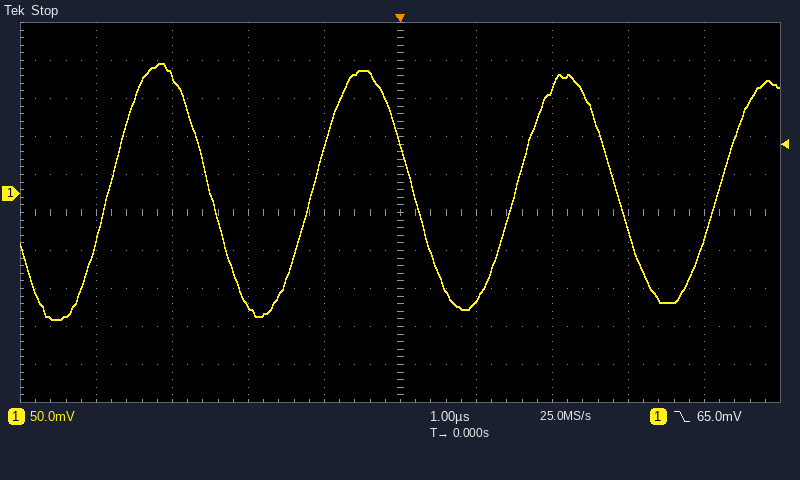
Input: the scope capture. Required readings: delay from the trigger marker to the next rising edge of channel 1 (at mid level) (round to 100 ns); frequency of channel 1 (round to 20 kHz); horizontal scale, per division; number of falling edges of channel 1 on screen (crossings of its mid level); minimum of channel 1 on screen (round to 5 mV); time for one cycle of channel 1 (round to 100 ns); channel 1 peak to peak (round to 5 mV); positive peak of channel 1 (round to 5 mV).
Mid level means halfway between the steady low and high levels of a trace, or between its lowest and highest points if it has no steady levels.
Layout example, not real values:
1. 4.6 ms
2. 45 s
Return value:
1. 1.5 µs
2. 380 kHz
3. 1 µs
4. 3
5. -165 mV
6. 2.7 µs
7. 335 mV
8. 170 mV
